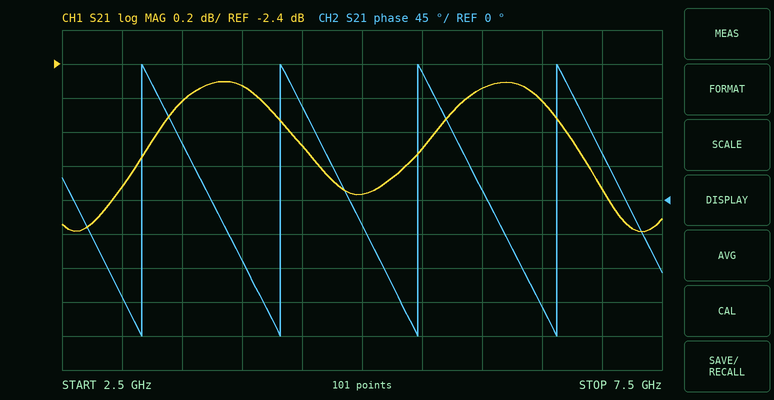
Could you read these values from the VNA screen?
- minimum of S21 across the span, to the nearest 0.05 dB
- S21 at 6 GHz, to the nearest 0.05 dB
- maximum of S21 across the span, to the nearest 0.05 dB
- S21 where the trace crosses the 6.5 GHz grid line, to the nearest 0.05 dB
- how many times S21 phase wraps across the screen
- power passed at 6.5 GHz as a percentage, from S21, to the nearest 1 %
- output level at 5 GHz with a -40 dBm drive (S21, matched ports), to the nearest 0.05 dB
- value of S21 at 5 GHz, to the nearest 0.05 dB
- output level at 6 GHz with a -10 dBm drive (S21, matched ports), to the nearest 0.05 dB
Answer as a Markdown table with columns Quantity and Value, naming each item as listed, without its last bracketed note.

| Quantity | Value |
|---|---|
| minimum of S21 across the span, to the nearest 0.05 dB | -3.40 dB |
| S21 at 6 GHz, to the nearest 0.05 dB | -2.55 dB |
| maximum of S21 across the span, to the nearest 0.05 dB | -2.50 dB |
| S21 where the trace crosses the 6.5 GHz grid line, to the nearest 0.05 dB | -2.60 dB |
| how many times S21 phase wraps across the screen | 4 |
| power passed at 6.5 GHz as a percentage, from S21, to the nearest 1 % | 55 % |
| output level at 5 GHz with a -40 dBm drive (S21, matched ports), to the nearest 0.05 dB | -43.15 dBm |
| value of S21 at 5 GHz, to the nearest 0.05 dB | -3.15 dB |
| output level at 6 GHz with a -10 dBm drive (S21, matched ports), to the nearest 0.05 dB | -12.55 dBm |
